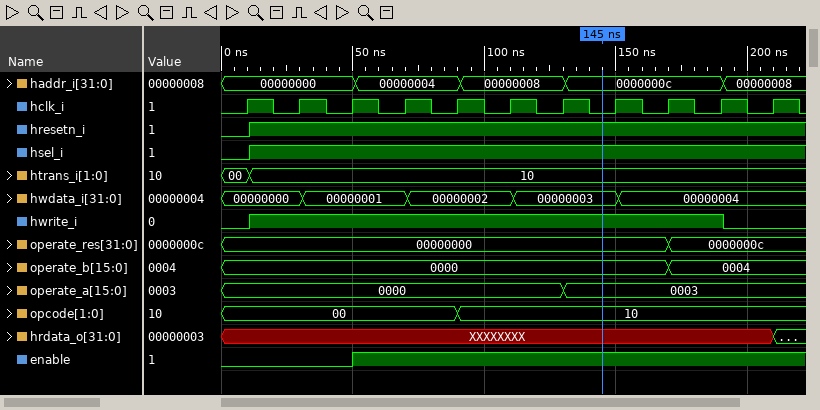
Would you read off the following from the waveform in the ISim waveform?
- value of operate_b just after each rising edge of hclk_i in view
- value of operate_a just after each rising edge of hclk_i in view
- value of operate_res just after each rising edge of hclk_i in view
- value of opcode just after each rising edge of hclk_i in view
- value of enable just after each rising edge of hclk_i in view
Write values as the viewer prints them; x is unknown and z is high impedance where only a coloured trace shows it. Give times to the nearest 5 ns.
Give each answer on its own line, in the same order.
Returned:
0000, 0000, 0000, 0000, 0000, 0000, 0000, 0000, 0004, 0004, 0004
0000, 0000, 0000, 0000, 0000, 0000, 0003, 0003, 0003, 0003, 0003
00000000, 00000000, 00000000, 00000000, 00000000, 00000000, 00000000, 00000000, 0000000c, 0000000c, 0000000c
00, 00, 00, 00, 10, 10, 10, 10, 10, 10, 10
0 0 1 1 1 1 1 1 1 1 1
